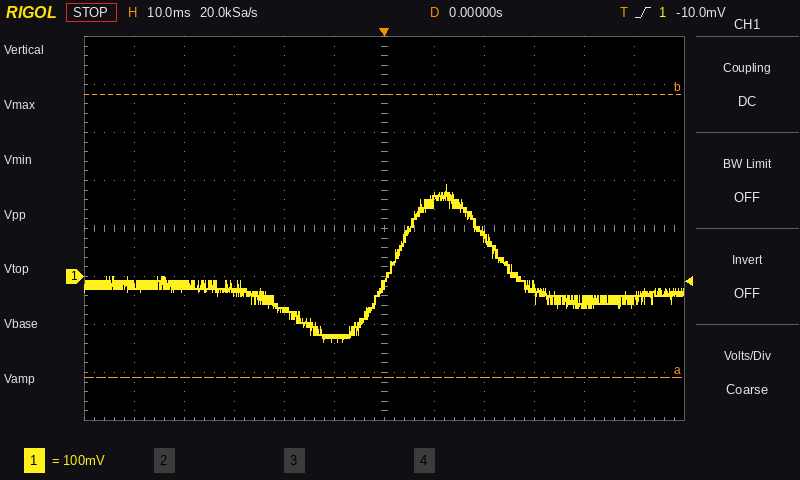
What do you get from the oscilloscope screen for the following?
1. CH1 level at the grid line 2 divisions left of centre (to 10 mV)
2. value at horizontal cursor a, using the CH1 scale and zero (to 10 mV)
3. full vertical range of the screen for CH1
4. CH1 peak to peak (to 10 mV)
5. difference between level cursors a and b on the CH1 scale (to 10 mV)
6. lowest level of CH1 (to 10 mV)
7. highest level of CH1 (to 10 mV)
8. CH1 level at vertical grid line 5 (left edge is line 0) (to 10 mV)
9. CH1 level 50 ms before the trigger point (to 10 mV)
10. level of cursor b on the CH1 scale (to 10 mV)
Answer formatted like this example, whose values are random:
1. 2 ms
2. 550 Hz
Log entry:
1. -70 mV
2. -210 mV
3. 800 mV
4. 330 mV
5. 590 mV
6. -140 mV
7. 190 mV
8. -130 mV
9. -20 mV
10. 380 mV
